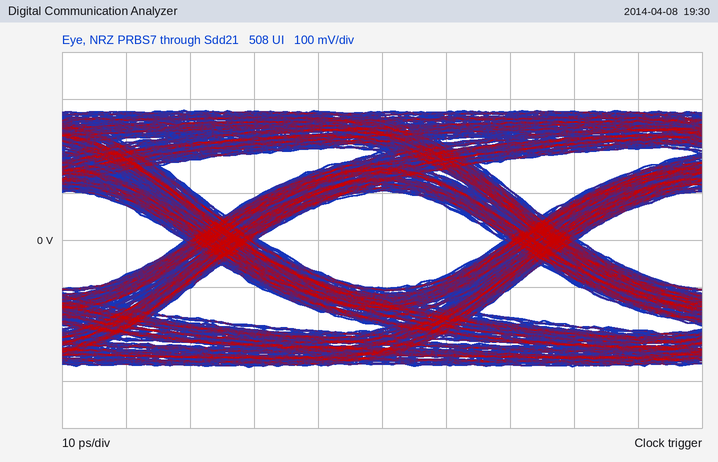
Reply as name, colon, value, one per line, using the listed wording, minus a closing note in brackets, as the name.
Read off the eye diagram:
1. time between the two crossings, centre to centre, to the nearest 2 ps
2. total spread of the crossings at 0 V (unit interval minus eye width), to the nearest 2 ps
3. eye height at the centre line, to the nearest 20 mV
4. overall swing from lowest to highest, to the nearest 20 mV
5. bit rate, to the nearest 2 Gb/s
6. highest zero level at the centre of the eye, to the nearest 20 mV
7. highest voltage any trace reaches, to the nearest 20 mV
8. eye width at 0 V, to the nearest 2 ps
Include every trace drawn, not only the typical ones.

time between the two crossings, centre to centre, to the nearest 2 ps: 50 ps
total spread of the crossings at 0 V (unit interval minus eye width), to the nearest 2 ps: 12 ps
eye height at the centre line, to the nearest 20 mV: 200 mV
overall swing from lowest to highest, to the nearest 20 mV: 540 mV
bit rate, to the nearest 2 Gb/s: 20 Gb/s
highest zero level at the centre of the eye, to the nearest 20 mV: -100 mV
highest voltage any trace reaches, to the nearest 20 mV: 280 mV
eye width at 0 V, to the nearest 2 ps: 38 ps
